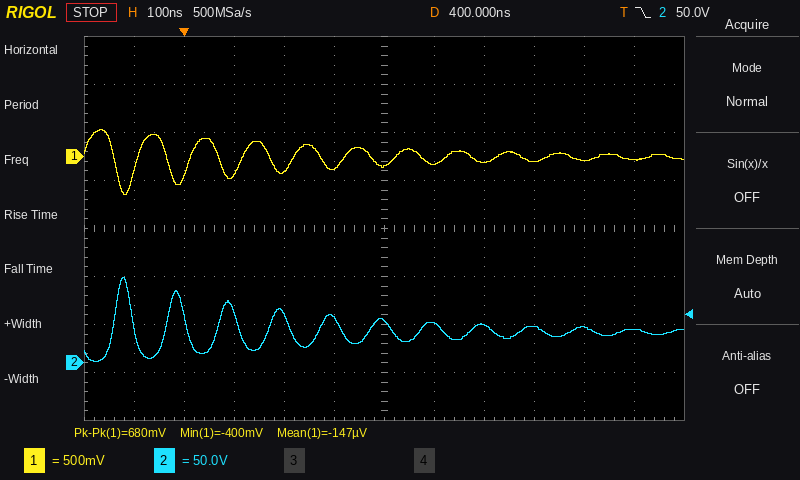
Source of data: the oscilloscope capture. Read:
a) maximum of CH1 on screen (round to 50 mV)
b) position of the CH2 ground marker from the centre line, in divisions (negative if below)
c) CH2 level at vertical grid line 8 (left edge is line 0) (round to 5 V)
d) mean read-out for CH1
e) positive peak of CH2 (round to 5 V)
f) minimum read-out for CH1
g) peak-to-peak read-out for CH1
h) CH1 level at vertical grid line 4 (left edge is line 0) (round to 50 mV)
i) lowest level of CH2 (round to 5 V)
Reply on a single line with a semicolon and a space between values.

300 mV; -2.8 div; 40 V; -147 µV; 90 V; -400 mV; 680 mV; -150 mV; 0 V
